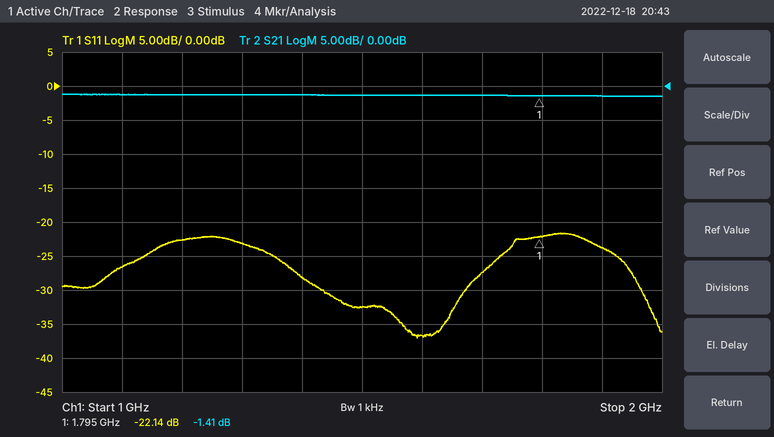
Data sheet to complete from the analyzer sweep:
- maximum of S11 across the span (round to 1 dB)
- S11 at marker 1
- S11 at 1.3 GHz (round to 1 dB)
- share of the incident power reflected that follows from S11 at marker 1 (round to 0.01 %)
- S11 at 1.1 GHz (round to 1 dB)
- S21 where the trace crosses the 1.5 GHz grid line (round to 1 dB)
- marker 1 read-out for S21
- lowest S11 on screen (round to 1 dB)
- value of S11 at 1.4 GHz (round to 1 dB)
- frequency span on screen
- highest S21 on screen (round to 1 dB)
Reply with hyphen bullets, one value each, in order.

- -22 dB
- -22.14 dB
- -23 dB
- 0.61 %
- -27 dB
- -1 dB
- -1.41 dB
- -37 dB
- -28 dB
- 1 GHz
- -1 dB
